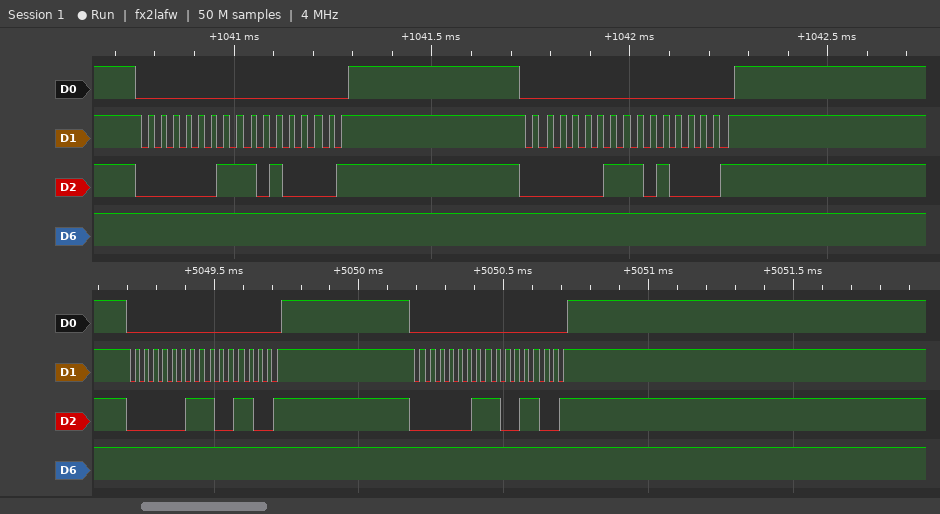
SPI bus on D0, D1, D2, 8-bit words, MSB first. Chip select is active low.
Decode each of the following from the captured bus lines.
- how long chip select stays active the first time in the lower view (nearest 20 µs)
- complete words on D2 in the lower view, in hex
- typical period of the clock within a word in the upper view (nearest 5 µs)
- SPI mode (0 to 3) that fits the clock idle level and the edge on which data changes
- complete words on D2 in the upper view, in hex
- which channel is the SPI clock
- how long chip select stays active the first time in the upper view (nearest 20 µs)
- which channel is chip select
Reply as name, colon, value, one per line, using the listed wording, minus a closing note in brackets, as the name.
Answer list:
how long chip select stays active the first time in the lower view: 540 µs
complete words on D2 in the lower view, in hex: 03, 99, 03, 99
typical period of the clock within a word in the upper view: 30 µs
SPI mode (0 to 3) that fits the clock idle level and the edge on which data changes: 3
complete words on D2 in the upper view, in hex: 03, A1, 03, A1
which channel is the SPI clock: D1
how long chip select stays active the first time in the upper view: 540 µs
which channel is chip select: D0
